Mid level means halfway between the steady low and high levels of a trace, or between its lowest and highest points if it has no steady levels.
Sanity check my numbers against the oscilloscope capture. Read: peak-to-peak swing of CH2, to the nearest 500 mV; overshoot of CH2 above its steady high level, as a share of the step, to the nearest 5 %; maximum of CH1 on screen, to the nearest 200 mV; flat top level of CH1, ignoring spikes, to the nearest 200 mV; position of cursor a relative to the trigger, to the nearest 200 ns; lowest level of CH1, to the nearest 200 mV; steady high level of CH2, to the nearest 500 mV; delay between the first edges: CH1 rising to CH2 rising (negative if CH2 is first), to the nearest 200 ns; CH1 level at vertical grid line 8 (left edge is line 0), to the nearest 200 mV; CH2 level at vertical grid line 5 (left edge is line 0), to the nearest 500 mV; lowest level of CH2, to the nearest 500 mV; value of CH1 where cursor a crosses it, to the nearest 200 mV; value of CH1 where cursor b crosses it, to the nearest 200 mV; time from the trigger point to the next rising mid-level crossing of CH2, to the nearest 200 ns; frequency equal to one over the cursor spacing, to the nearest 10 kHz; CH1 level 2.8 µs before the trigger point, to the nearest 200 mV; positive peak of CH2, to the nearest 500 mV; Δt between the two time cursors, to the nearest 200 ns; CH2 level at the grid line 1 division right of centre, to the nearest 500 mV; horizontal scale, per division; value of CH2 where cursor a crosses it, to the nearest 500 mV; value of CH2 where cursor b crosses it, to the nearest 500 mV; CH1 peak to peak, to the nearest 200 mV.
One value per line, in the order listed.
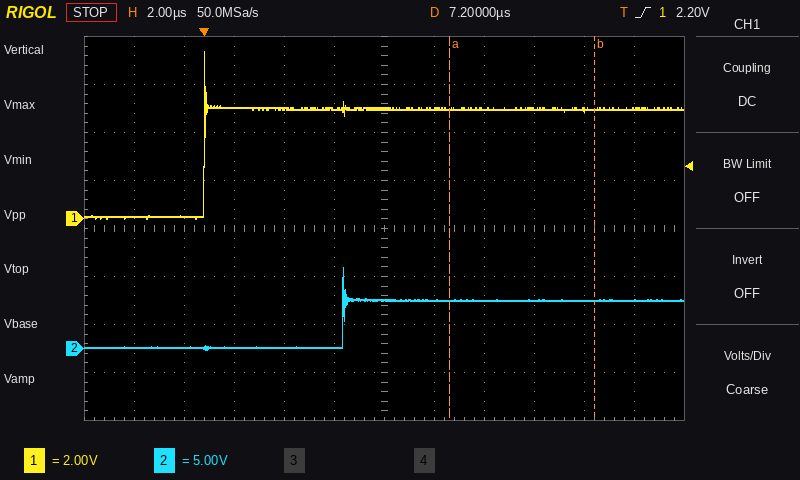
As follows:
8.5 V
70 %
7.0 V
4.6 V
+9.8 µs
0.0 V
5.0 V
+5.6 µs
4.6 V
0.0 V
0.0 V
4.6 V
4.6 V
5.6 µs
170 kHz
0.0 V
8.5 V
5.8 µs
5.0 V
2 µs
5.0 V
5.0 V
7.0 V
